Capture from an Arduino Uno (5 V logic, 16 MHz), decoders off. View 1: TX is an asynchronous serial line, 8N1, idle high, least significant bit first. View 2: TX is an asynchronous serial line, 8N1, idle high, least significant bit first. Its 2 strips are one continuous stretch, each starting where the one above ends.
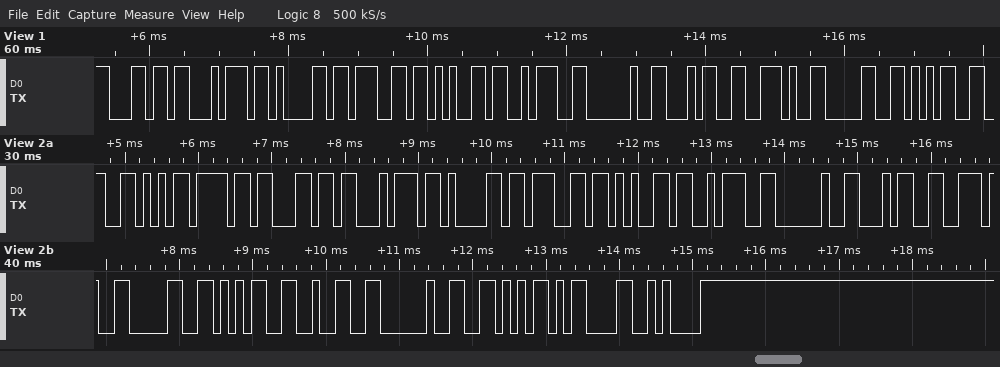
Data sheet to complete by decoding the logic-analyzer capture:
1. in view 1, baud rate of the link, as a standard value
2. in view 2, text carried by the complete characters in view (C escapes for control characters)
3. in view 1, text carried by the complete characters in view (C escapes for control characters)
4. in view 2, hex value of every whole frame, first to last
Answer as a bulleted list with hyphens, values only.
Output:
- 9600 baud
- "Voltage: 4.052 V\r\n"
- "ltage: 4.05"
- 56 6F 6C 74 61 67 65 3A 20 34 2E 30 35 32 20 56 0D 0A
